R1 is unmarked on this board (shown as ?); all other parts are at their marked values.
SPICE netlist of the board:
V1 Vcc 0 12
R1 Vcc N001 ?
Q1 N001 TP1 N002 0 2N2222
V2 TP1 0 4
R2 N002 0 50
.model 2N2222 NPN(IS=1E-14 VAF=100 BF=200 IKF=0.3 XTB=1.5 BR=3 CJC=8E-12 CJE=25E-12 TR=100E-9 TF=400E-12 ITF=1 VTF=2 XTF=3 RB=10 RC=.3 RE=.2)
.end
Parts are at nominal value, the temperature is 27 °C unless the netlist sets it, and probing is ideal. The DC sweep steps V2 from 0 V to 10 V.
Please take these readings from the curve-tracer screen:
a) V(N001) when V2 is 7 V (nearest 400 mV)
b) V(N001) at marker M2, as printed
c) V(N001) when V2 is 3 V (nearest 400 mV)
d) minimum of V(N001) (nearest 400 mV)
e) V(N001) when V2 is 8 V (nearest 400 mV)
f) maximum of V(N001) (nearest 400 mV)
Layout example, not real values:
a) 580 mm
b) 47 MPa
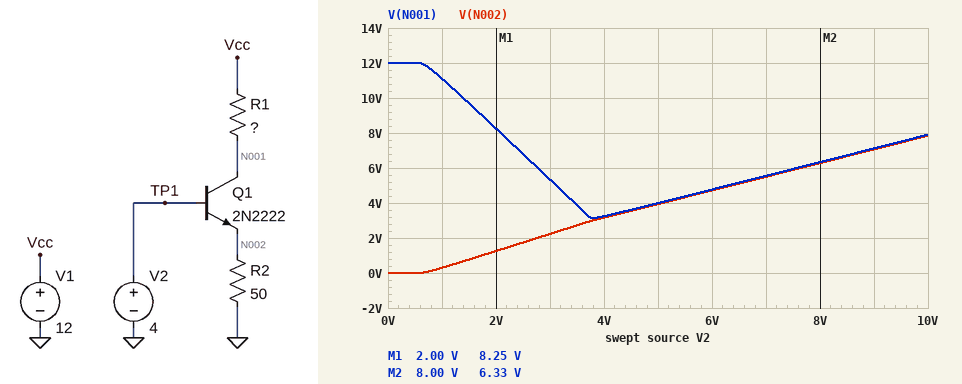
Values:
a) 5.6 V
b) 6.33 V
c) 5.2 V
d) 3.2 V
e) 6.4 V
f) 12.0 V
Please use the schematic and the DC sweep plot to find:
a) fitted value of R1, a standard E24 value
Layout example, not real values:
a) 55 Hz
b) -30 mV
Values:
a) 150 Ω
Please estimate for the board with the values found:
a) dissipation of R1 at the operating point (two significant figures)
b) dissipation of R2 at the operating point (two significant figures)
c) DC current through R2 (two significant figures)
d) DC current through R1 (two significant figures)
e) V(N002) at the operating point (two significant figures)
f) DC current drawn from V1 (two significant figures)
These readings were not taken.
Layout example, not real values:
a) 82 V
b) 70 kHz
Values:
a) 510 mW
b) 200 mW
c) 63 mA
d) 58 mA
e) 3.2 V
f) 58 mA
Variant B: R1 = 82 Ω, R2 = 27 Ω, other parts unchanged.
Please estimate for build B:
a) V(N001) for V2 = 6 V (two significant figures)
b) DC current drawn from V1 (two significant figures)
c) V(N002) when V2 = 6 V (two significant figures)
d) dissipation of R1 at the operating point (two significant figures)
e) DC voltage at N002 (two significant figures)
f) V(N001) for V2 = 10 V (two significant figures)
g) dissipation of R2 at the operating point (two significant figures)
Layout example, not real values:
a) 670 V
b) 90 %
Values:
a) 4.5 V
b) 110 mA
c) 4.4 V
d) 940 mW
e) 3.1 V
f) 7.2 V
g) 360 mW
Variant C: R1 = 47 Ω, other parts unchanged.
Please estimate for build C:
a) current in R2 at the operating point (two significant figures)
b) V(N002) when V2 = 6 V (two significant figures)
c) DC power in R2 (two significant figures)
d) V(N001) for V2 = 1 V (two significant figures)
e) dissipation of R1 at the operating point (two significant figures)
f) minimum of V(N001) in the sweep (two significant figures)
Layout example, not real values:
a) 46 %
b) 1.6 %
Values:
a) 64 mA
b) 5.2 V
c) 210 mW
d) 12 V
e) 190 mW
f) 6.3 V
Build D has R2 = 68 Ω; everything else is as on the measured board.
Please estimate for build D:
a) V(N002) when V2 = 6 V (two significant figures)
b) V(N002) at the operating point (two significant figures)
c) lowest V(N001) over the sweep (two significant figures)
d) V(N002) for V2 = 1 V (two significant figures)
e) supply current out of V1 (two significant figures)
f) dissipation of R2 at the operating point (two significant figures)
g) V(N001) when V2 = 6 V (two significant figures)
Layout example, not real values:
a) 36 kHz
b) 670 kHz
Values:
a) 4.9 V
b) 3.2 V
c) 3.9 V
d) 310 mV
e) 47 mA
f) 150 mW
g) 5.0 V
